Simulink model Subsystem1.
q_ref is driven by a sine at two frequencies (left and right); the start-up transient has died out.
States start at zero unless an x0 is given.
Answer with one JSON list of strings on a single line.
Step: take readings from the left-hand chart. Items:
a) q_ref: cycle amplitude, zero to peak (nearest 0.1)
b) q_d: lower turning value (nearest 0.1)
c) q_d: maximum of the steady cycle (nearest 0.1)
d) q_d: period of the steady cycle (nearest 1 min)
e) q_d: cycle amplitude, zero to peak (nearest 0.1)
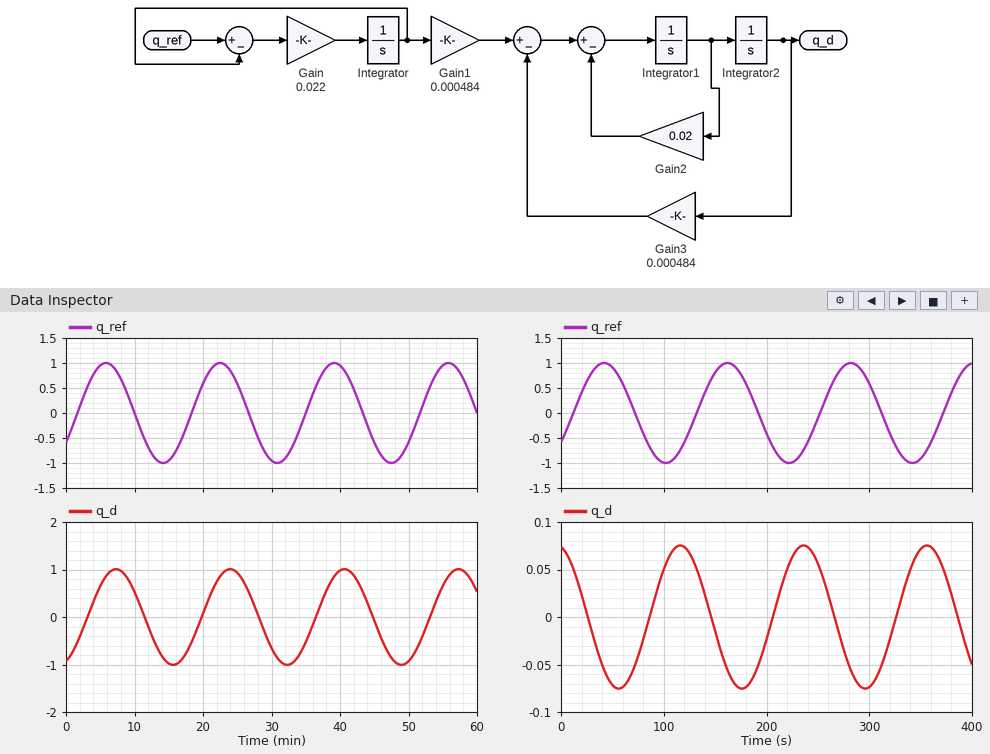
["1.0", "-1.0", "1.0", "17 min", "1.0"]
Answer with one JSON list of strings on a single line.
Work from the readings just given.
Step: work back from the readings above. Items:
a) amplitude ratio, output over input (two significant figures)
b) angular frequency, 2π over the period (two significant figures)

["1.0", "0.37 rad/min"]
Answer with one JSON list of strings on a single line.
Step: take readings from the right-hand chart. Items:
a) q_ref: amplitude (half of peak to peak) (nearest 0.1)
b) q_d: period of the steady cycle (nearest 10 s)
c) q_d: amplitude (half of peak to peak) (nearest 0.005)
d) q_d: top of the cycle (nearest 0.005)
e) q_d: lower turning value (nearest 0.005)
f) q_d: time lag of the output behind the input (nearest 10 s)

["1.0", "120 s", "0.075", "0.075", "-0.075", "70 s"]
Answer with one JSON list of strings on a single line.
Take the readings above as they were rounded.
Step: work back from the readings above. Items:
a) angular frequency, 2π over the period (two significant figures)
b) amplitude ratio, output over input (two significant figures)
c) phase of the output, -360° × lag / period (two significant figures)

["0.052 rad/s", "0.075", "-210°"]
